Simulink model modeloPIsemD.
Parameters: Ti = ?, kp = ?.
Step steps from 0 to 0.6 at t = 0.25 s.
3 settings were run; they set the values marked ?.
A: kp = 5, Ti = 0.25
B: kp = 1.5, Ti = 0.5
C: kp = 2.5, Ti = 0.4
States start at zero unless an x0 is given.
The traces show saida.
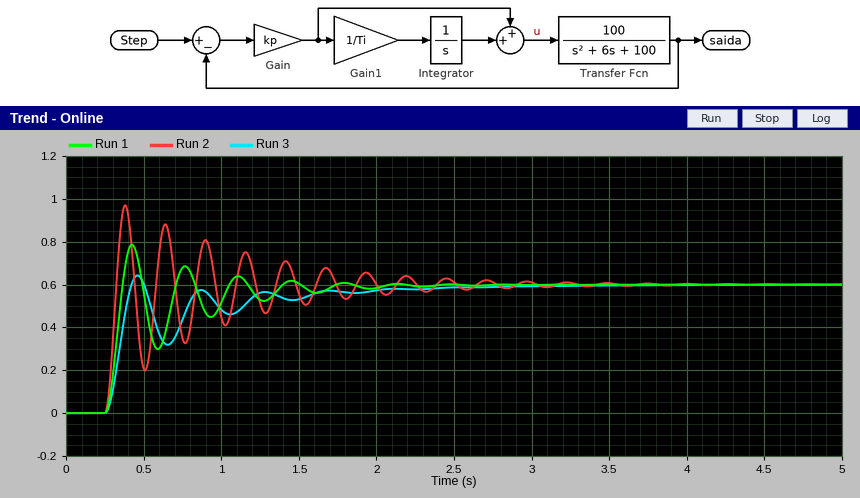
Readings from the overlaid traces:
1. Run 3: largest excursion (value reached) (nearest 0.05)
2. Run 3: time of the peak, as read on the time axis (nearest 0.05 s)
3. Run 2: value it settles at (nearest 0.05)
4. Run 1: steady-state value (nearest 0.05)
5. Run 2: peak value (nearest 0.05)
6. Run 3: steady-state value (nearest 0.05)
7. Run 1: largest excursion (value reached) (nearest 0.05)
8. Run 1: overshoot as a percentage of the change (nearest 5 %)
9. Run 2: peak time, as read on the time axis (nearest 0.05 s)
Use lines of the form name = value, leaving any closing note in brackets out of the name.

Run 3: largest excursion (value reached) = 0.65
Run 3: time of the peak, as read on the time axis = 0.45 s
Run 2: value it settles at = 0.60
Run 1: steady-state value = 0.60
Run 2: peak value = 0.95
Run 3: steady-state value = 0.60
Run 1: largest excursion (value reached) = 0.80
Run 1: overshoot as a percentage of the change = 30 %
Run 2: peak time, as read on the time axis = 0.40 s
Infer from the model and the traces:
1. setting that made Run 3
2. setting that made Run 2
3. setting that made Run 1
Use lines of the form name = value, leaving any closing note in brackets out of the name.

setting that made Run 3 = B
setting that made Run 2 = A
setting that made Run 1 = C
